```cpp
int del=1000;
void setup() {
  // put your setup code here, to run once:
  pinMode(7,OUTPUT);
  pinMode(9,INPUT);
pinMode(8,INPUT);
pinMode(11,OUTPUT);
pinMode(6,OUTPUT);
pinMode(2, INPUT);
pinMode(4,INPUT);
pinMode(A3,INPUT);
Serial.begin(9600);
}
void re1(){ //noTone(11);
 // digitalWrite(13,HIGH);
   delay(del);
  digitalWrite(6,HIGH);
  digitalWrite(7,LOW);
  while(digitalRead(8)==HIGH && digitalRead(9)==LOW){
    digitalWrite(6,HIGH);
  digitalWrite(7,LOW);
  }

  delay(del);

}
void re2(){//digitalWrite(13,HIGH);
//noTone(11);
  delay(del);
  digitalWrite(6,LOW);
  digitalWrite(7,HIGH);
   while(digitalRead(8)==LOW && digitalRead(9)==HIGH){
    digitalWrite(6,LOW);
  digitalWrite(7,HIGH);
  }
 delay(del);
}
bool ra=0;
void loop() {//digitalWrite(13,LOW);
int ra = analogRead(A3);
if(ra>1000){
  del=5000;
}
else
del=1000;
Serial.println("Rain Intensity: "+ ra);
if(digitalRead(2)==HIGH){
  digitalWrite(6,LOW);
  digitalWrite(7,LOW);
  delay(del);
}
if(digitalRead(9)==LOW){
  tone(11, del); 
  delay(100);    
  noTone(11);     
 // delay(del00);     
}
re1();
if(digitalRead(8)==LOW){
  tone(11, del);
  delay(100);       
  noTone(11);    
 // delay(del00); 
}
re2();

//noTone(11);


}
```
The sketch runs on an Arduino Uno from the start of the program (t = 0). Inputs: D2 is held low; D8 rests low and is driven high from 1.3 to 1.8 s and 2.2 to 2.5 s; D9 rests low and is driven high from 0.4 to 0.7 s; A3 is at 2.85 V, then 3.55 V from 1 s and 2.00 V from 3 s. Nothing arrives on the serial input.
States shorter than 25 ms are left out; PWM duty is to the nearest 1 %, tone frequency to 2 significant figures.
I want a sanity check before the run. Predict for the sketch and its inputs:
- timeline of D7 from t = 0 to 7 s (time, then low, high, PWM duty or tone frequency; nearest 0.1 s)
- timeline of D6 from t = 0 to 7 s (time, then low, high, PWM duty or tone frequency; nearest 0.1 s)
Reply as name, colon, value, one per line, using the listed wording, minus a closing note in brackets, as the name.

timeline of D7 from t = 0 to 7 s: 0 s low; 3.2 s high; 5.3 s low
timeline of D6 from t = 0 to 7 s: 0 s low; 1.1 s high; 3.2 s low; 5.3 s high
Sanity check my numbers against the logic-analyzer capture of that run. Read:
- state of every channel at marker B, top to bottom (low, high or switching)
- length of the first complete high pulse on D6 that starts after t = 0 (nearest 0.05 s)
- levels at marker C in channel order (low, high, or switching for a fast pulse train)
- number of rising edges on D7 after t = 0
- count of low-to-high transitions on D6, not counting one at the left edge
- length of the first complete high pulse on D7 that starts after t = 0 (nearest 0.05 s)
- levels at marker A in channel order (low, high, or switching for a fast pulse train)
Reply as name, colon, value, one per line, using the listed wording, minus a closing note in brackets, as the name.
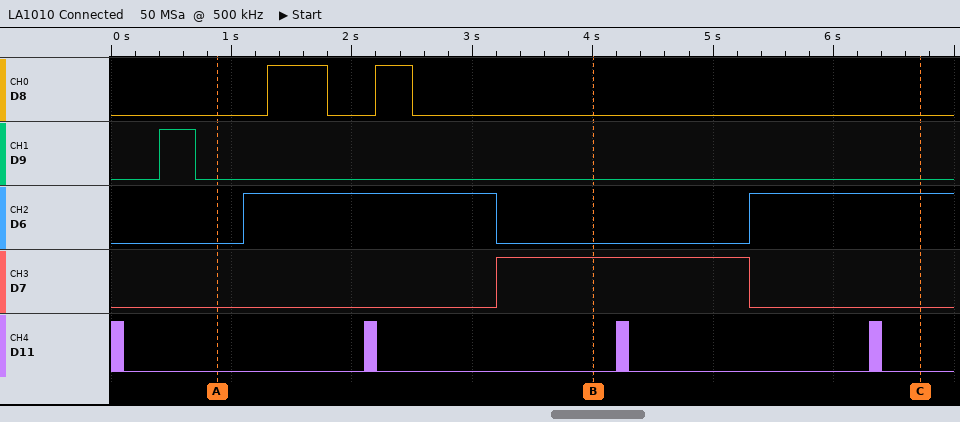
state of every channel at marker B, top to bottom: D8 low, D9 low, D6 low, D7 high, D11 low
length of the first complete high pulse on D6 that starts after t = 0: 2.10 s
levels at marker C in channel order: D8 low, D9 low, D6 high, D7 low, D11 low
number of rising edges on D7 after t = 0: 1
count of low-to-high transitions on D6, not counting one at the left edge: 2
length of the first complete high pulse on D7 that starts after t = 0: 2.10 s
levels at marker A in channel order: D8 low, D9 low, D6 low, D7 low, D11 low
